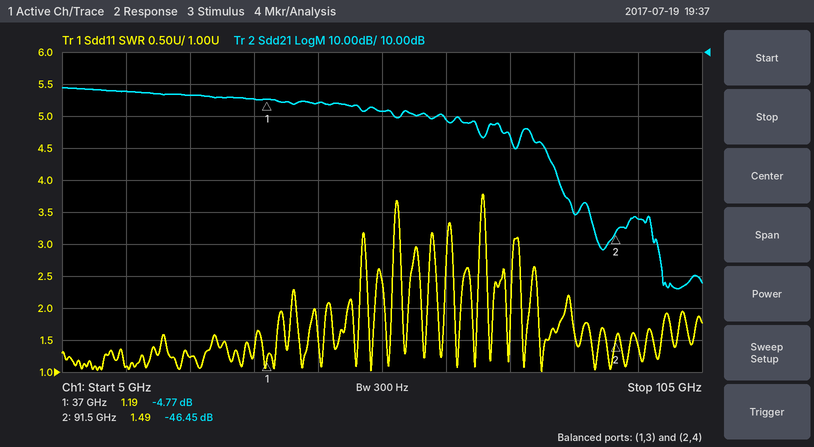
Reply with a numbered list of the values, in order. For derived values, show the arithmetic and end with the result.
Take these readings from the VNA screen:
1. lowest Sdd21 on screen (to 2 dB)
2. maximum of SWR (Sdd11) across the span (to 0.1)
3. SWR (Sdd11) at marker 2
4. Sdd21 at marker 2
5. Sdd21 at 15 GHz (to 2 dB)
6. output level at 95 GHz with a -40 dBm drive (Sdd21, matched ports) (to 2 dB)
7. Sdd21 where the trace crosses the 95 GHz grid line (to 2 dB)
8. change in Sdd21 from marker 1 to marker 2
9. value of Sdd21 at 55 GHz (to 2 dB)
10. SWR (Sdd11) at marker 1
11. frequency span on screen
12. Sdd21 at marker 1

1. -64 dB
2. 3.8
3. 1.49
4. -46.45 dB
5. -2 dB
6. -40 dBm + (-42 dB) = -82 dBm
7. -42 dB
8. -46.45 − (-4.77) = -41.68 dB
9. -8 dB
10. 1.19
11. 100 GHz
12. -4.77 dB
